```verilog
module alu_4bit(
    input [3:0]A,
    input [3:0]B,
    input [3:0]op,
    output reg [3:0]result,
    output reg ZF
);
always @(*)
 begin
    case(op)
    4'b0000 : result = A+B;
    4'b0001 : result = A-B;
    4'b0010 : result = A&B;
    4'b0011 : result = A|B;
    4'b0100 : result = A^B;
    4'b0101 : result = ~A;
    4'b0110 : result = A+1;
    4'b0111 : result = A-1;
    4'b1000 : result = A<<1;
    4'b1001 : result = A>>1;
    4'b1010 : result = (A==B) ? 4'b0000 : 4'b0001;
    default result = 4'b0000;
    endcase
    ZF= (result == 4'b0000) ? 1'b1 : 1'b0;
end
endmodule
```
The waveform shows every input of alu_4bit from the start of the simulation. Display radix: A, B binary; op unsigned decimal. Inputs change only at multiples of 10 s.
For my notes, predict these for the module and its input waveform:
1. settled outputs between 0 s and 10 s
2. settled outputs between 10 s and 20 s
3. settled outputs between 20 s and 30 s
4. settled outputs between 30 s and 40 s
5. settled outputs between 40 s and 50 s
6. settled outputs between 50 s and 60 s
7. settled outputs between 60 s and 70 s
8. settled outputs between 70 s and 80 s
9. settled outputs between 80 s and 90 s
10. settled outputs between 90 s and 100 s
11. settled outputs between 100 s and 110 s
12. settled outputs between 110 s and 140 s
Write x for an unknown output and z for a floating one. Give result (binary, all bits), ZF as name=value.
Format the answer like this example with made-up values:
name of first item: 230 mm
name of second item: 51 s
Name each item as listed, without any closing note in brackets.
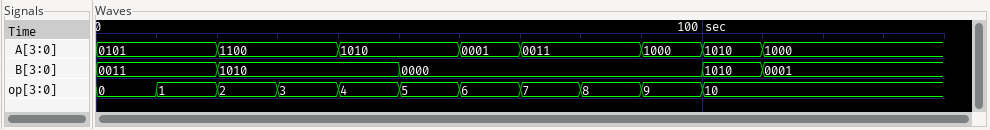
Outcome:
settled outputs between 0 s and 10 s: result=1000, ZF=0
settled outputs between 10 s and 20 s: result=0010, ZF=0
settled outputs between 20 s and 30 s: result=1000, ZF=0
settled outputs between 30 s and 40 s: result=1110, ZF=0
settled outputs between 40 s and 50 s: result=0000, ZF=1
settled outputs between 50 s and 60 s: result=0101, ZF=0
settled outputs between 60 s and 70 s: result=0010, ZF=0
settled outputs between 70 s and 80 s: result=0010, ZF=0
settled outputs between 80 s and 90 s: result=0110, ZF=0
settled outputs between 90 s and 100 s: result=0100, ZF=0
settled outputs between 100 s and 110 s: result=0000, ZF=1
settled outputs between 110 s and 140 s: result=0001, ZF=0
